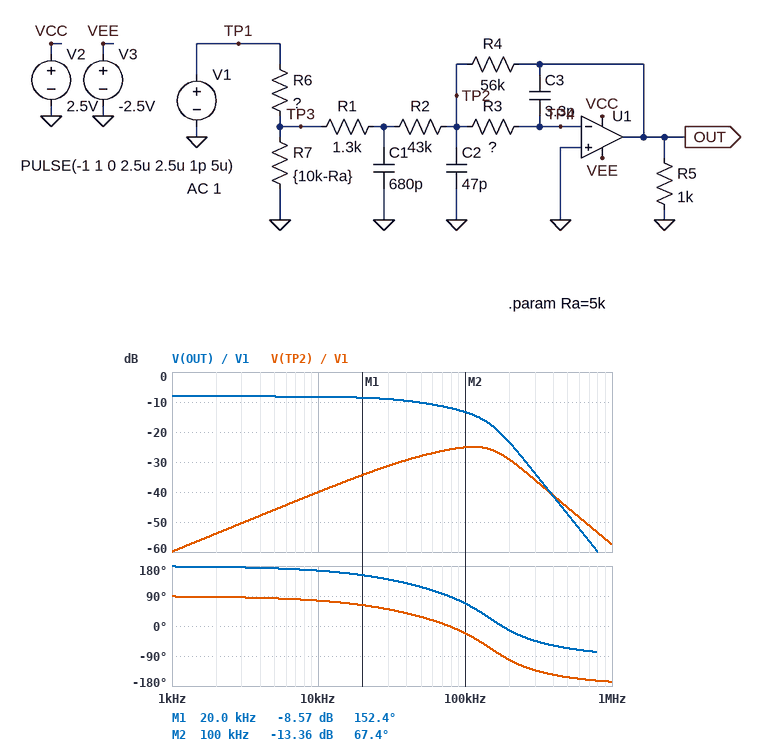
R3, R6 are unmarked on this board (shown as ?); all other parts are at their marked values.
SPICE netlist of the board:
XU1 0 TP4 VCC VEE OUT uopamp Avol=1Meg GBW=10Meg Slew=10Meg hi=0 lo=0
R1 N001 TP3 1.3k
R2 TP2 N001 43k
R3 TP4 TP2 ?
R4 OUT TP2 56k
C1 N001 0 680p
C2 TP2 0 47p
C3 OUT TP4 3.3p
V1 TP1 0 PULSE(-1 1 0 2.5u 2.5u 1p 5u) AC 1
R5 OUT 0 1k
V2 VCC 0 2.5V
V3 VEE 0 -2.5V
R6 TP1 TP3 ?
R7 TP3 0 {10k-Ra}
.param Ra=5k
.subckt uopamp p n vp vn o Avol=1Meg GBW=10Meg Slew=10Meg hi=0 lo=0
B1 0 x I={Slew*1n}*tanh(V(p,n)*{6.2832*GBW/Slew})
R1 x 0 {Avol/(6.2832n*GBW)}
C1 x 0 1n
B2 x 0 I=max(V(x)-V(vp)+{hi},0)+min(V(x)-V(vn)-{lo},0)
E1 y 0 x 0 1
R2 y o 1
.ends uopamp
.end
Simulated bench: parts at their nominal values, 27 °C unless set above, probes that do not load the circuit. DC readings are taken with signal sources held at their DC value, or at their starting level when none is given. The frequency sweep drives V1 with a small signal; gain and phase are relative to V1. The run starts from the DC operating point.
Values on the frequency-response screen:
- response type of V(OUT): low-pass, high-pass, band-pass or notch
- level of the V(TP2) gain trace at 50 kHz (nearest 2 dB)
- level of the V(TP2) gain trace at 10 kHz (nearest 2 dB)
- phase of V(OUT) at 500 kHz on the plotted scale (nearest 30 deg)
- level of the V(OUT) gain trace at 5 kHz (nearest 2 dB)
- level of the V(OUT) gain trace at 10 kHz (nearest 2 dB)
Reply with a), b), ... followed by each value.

a) low-pass
b) -28 dB
c) -40 dB
d) -60 deg
e) -8 dB
f) -8 dB
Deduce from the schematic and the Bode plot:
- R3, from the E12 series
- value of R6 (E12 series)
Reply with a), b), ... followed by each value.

a) 120 kΩ
b) 10 kΩ
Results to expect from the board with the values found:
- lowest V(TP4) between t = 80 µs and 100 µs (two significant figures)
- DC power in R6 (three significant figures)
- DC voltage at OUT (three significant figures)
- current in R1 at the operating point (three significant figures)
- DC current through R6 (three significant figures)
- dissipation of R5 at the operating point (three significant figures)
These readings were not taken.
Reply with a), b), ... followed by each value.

a) -1.1 mV
b) 47.6 µW
c) 392 mV
d) 7.00 µA
e) 69.0 µA
f) 154 µW
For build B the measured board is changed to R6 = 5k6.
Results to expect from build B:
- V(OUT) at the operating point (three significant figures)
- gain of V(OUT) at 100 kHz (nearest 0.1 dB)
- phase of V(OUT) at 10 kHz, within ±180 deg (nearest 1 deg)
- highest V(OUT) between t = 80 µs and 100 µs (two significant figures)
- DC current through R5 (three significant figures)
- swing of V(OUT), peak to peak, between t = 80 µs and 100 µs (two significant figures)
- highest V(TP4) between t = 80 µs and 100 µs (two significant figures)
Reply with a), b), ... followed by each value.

a) 563 mV
b) -9.3 dB
c) 167 deg
d) 89 mV
e) 563 µA
f) 180 mV
g) 1.8 mV
